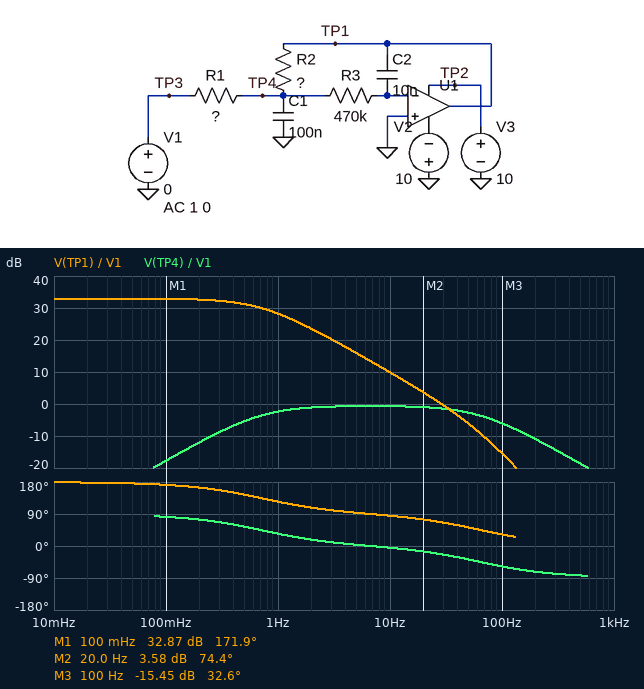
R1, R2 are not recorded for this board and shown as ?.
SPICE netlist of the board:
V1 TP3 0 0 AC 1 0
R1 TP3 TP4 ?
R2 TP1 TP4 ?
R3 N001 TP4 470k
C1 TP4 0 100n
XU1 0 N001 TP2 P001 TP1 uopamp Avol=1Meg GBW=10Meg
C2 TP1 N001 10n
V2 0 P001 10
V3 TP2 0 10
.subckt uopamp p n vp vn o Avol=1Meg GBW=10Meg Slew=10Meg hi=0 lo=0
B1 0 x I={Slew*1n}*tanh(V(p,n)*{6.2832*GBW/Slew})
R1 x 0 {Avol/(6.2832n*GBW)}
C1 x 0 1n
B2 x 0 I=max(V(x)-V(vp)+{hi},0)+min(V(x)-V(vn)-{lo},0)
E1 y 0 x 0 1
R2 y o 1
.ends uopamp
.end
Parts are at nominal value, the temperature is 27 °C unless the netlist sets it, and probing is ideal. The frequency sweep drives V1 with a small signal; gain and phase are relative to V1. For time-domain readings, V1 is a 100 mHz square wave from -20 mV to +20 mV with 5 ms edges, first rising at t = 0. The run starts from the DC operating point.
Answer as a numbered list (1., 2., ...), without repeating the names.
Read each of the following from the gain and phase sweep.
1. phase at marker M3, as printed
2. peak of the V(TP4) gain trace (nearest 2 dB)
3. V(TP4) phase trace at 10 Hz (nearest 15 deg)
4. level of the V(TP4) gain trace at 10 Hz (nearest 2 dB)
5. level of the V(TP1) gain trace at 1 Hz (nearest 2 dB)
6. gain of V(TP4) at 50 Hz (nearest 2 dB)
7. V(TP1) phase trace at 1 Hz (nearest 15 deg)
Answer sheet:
1. 32.6 deg
2. 0 dB
3. 0 deg
4. 0 dB
5. 28 dB
6. -2 dB
7. 120 deg
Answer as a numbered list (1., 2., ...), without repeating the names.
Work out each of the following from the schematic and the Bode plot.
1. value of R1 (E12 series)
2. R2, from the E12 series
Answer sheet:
1. 27 kΩ
2. 1.2 MΩ
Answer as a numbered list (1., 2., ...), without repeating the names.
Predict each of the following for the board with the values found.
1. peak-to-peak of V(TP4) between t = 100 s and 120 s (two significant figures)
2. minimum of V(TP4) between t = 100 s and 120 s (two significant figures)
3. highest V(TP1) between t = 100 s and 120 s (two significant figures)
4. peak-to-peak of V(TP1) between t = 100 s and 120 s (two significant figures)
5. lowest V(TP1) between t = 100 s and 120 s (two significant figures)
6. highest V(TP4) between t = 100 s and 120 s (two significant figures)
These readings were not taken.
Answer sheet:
1. 71 mV
2. -36 mV
3. 890 mV
4. 1.8 V
5. -890 mV
6. 36 mV
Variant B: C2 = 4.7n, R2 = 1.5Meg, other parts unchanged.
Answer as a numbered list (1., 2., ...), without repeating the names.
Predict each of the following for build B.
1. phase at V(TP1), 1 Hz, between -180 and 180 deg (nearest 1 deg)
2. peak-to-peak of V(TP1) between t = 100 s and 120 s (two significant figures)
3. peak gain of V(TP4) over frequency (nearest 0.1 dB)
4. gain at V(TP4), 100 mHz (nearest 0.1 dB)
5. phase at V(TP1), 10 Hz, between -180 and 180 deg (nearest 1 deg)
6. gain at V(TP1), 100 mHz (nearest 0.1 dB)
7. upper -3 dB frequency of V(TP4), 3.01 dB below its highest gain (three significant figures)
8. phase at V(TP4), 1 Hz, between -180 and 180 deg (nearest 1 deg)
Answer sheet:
1. 140 deg
2. 2.2 V
3. -0.6 dB
4. -22.3 dB
5. 88 deg
6. 34.9 dB
7. 64.6 Hz
8. 50 deg
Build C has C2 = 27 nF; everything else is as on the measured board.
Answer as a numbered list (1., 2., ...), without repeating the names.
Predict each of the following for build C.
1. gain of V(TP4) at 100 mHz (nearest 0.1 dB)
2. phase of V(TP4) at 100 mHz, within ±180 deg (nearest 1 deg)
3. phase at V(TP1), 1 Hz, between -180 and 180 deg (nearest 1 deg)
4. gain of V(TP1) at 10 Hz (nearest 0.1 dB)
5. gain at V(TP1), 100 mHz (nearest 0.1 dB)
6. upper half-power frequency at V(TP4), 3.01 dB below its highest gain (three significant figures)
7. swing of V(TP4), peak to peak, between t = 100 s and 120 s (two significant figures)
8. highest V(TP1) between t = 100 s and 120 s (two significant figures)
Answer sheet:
1. -9.6 dB
2. 69 deg
3. 104 deg
4. 1.2 dB
5. 32.4 dB
6. 63.9 Hz
7. 73 mV
8. 890 mV
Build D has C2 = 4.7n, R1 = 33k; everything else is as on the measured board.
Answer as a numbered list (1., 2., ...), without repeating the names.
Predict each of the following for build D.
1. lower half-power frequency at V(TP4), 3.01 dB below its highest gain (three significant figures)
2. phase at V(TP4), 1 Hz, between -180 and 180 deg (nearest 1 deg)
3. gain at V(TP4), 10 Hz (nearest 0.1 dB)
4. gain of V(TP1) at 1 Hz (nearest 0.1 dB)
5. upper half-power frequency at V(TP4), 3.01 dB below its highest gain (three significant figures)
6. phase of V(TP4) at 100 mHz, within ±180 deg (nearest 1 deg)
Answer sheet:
1. 1.75 Hz
2. 61 deg
3. -0.8 dB
4. 30.1 dB
5. 54.7 Hz
6. 87 deg
